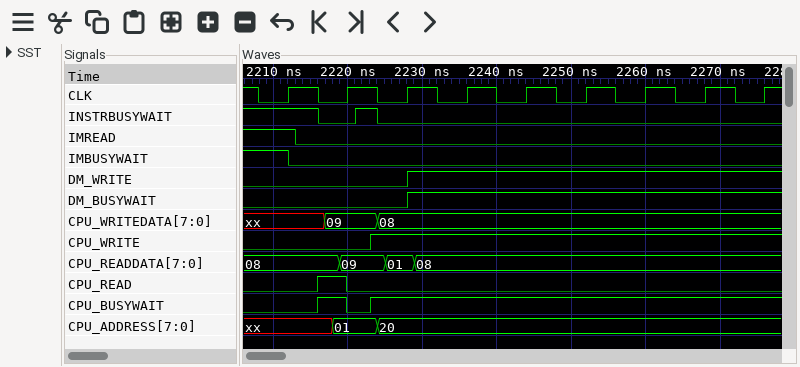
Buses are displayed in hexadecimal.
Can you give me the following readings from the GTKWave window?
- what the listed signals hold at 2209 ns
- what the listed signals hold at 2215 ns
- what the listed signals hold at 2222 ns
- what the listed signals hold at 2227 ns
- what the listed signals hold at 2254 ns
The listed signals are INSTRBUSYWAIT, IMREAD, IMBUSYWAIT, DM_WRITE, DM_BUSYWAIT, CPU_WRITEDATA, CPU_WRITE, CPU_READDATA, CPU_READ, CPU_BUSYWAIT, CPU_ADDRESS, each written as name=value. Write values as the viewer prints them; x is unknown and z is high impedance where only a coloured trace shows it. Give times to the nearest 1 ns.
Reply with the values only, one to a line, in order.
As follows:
INSTRBUSYWAIT=1, IMREAD=1, IMBUSYWAIT=1, DM_WRITE=0, DM_BUSYWAIT=0, CPU_WRITEDATA=xx, CPU_WRITE=0, CPU_READDATA=08, CPU_READ=0, CPU_BUSYWAIT=0, CPU_ADDRESS=xx
INSTRBUSYWAIT=1, IMREAD=0, IMBUSYWAIT=0, DM_WRITE=0, DM_BUSYWAIT=0, CPU_WRITEDATA=xx, CPU_WRITE=0, CPU_READDATA=08, CPU_READ=0, CPU_BUSYWAIT=0, CPU_ADDRESS=xx
INSTRBUSYWAIT=1, IMREAD=0, IMBUSYWAIT=0, DM_WRITE=0, DM_BUSYWAIT=0, CPU_WRITEDATA=09, CPU_WRITE=0, CPU_READDATA=09, CPU_READ=0, CPU_BUSYWAIT=0, CPU_ADDRESS=01
INSTRBUSYWAIT=0, IMREAD=0, IMBUSYWAIT=0, DM_WRITE=0, DM_BUSYWAIT=0, CPU_WRITEDATA=08, CPU_WRITE=1, CPU_READDATA=01, CPU_READ=0, CPU_BUSYWAIT=1, CPU_ADDRESS=20
INSTRBUSYWAIT=0, IMREAD=0, IMBUSYWAIT=0, DM_WRITE=1, DM_BUSYWAIT=1, CPU_WRITEDATA=08, CPU_WRITE=1, CPU_READDATA=08, CPU_READ=0, CPU_BUSYWAIT=1, CPU_ADDRESS=20
